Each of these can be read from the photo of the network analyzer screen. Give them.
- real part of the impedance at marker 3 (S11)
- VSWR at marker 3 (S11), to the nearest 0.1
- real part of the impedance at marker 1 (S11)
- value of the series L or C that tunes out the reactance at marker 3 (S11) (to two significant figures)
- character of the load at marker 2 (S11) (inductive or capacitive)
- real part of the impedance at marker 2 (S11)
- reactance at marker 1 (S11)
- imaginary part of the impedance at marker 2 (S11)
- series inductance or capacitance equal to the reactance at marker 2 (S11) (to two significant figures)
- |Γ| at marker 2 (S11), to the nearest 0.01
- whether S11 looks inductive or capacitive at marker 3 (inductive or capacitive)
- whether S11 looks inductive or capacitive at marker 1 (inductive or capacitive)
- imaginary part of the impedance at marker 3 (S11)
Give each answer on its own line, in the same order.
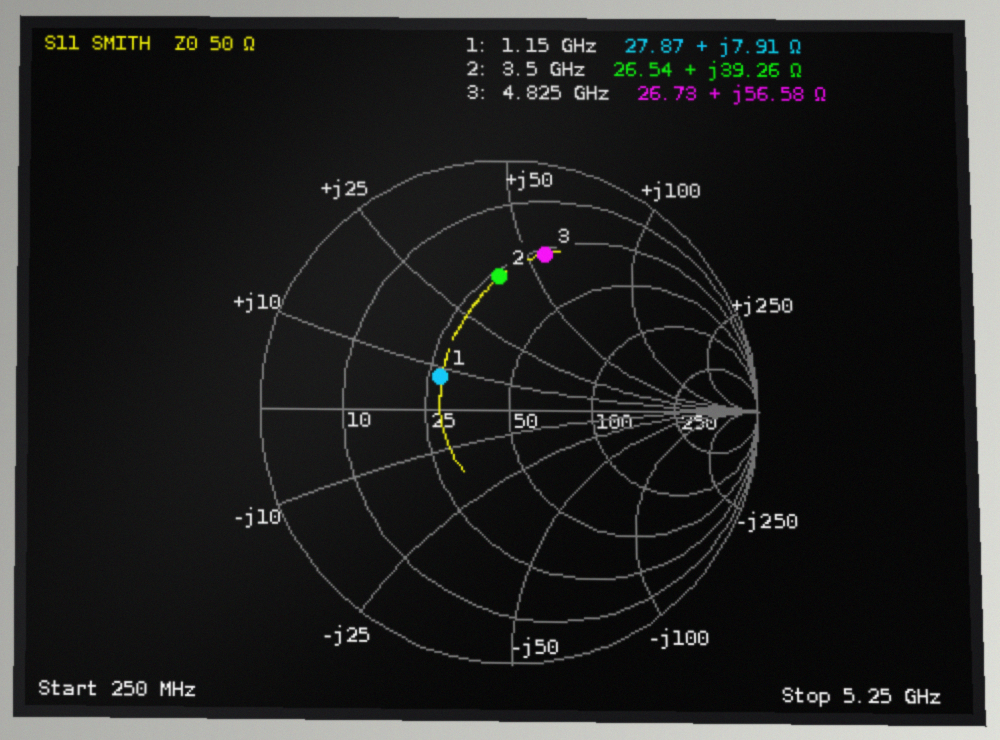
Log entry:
26.73 Ω
4.6
27.87 Ω
580 fF
inductive
26.54 Ω
+7.91 Ω
+39.26 Ω
1.8 nH
0.53
inductive
inductive
+56.58 Ω
